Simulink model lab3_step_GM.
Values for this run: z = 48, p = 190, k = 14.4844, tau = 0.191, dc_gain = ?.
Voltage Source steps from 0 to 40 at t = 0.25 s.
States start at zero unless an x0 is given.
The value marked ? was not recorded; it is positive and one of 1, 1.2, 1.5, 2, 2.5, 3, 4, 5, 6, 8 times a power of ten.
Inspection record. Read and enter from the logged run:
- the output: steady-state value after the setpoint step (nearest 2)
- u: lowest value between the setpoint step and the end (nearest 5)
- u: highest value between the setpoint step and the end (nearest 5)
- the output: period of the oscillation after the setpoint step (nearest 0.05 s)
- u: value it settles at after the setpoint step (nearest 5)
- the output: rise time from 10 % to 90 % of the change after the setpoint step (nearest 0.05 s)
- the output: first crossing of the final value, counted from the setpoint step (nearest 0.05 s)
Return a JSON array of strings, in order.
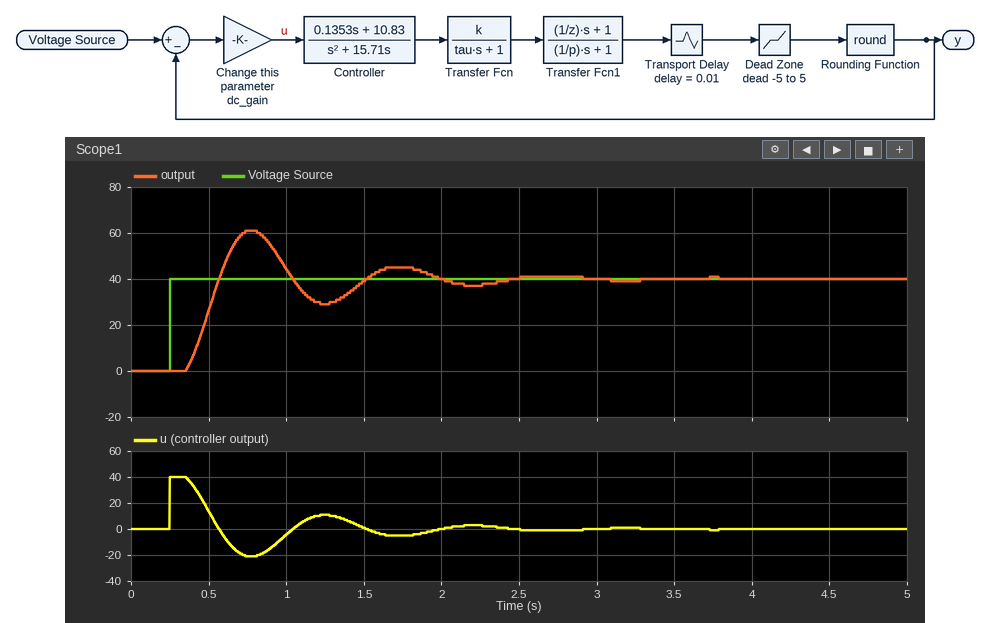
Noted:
["40", "-20", "40", "0.95 s", "0", "0.15 s", "0.30 s"]
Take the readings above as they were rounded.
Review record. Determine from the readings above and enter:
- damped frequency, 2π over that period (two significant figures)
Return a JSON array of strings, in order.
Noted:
["6.6 rad/s"]
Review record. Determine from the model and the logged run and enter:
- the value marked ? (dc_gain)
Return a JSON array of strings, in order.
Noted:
["1"]
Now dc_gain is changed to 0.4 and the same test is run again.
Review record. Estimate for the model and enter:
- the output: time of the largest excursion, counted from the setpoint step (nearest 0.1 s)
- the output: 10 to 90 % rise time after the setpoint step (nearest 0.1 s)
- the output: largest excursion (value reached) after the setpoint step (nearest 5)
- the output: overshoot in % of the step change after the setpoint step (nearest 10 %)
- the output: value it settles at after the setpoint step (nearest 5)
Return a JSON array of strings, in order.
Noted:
["0.8 s", "0.3 s", "50", "20 %", "40"]
